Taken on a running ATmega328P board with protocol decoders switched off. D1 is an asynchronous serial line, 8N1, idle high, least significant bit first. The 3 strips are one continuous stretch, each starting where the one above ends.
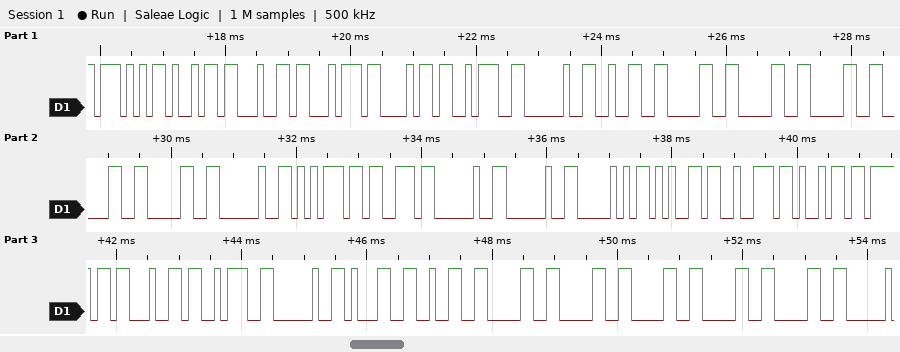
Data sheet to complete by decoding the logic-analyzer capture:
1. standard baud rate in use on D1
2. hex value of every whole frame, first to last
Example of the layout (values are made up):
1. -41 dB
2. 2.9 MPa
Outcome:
1. 9600 baud
2. 0x57 0x69 0x64 0x74 0x68 0x3A 0x20 0x32 0x30 0x30 0x30 0x30 0x30 0x20 0x75 0x73 0x20 0x20 0x50 0x65 0x72 0x69 0x6F 0x64 0x3A 0x20 0x31 0x32 0x30 0x30 0x30 0x30 0x30
